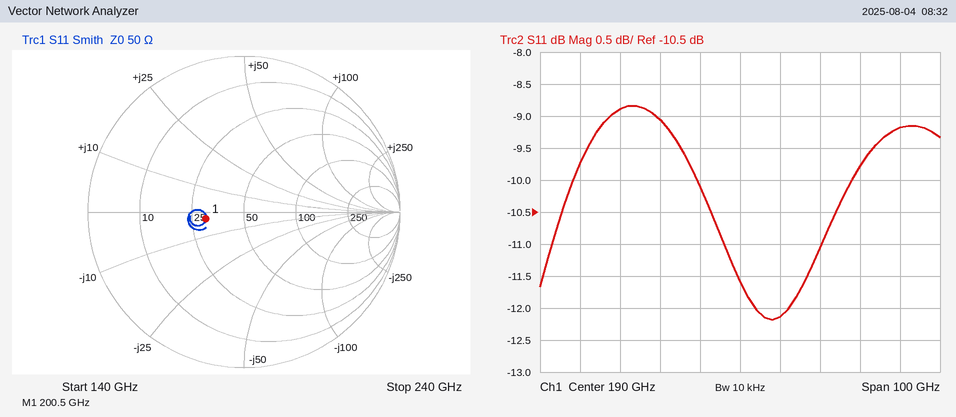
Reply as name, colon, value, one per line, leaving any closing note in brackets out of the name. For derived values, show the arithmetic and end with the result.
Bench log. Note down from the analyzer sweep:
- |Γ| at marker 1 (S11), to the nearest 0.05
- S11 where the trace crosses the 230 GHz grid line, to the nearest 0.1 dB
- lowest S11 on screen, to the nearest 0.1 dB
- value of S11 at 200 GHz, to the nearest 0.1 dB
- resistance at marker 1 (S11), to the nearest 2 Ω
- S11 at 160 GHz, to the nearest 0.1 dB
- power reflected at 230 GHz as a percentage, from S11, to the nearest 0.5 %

|Γ| at marker 1 (S11), to the nearest 0.05: 0.25
S11 where the trace crosses the 230 GHz grid line, to the nearest 0.1 dB: -9.2 dB
lowest S11 on screen, to the nearest 0.1 dB: -12.2 dB
value of S11 at 200 GHz, to the nearest 0.1 dB: -12.1 dB
resistance at marker 1 (S11), to the nearest 2 Ω: 30 Ω
S11 at 160 GHz, to the nearest 0.1 dB: -8.9 dB
power reflected at 230 GHz as a percentage, from S11, to the nearest 0.5 %: 10^(-9.2/10) ≈ 12.0 %
